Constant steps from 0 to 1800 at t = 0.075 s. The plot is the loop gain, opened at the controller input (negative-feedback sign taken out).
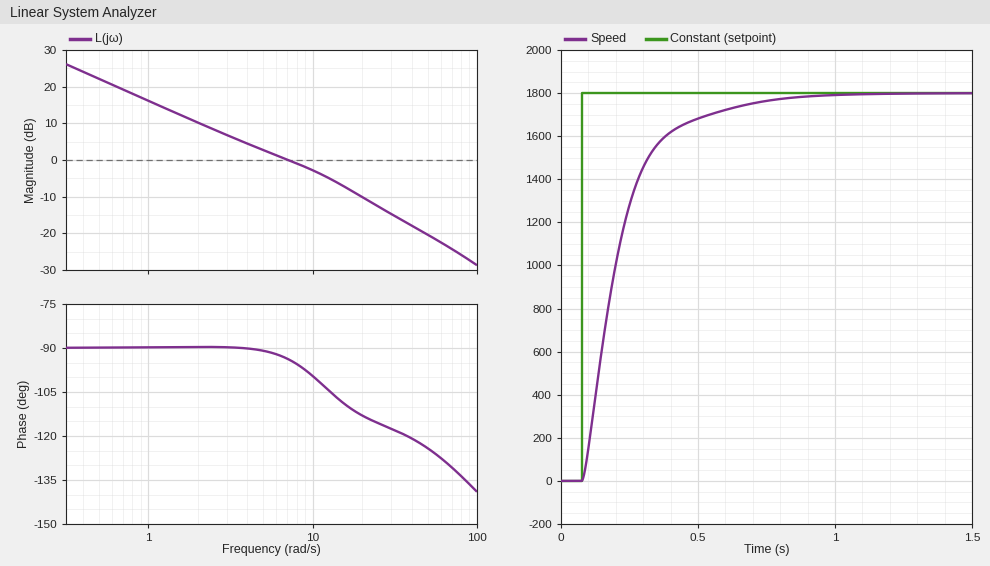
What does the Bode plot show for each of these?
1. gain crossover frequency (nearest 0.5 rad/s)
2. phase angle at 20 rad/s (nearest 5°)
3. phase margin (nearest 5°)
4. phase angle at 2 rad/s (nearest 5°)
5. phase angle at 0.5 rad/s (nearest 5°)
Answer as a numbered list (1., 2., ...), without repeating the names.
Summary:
1. 7.0 rad/s
2. -115°
3. 85°
4. -90°
5. -90°
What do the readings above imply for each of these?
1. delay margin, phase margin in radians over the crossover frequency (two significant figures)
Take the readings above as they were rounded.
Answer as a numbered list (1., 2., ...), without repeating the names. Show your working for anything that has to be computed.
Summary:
1. 85 × π / 180 / 7 = 0.21 s
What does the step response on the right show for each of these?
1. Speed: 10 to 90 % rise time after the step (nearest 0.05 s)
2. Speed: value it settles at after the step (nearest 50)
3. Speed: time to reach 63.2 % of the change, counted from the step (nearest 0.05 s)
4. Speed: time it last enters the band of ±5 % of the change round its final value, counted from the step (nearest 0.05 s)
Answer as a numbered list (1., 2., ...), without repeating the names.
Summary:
1. 0.30 s
2. 1800
3. 0.15 s
4. 0.50 s
